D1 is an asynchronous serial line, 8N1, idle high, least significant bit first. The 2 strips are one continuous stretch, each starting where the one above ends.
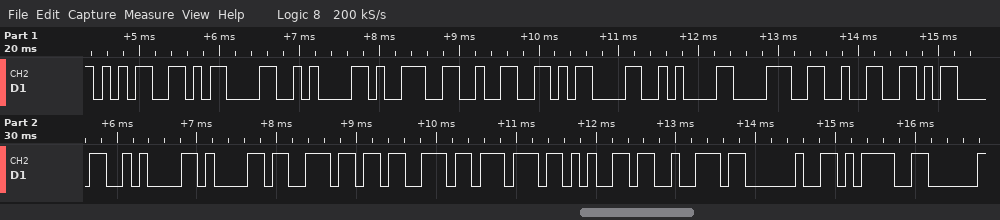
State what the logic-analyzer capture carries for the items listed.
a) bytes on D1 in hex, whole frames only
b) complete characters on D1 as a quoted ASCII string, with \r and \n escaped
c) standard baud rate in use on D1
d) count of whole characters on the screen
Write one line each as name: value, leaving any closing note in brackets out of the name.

bytes on D1 in hex, whole frames only: 0x35 0x0D 0x0A 0x39 0x32 0x0D 0x0A 0x38 0x32 0x0D 0x0A 0x61 0x6E 0x73 0x77 0x65 0x72 0x20 0x3D
complete characters on D1 as a quoted ASCII string, with \r and \n escaped: "5\r\n92\r\n82\r\nanswer ="
standard baud rate in use on D1: 9600 baud
count of whole characters on the screen: 19
